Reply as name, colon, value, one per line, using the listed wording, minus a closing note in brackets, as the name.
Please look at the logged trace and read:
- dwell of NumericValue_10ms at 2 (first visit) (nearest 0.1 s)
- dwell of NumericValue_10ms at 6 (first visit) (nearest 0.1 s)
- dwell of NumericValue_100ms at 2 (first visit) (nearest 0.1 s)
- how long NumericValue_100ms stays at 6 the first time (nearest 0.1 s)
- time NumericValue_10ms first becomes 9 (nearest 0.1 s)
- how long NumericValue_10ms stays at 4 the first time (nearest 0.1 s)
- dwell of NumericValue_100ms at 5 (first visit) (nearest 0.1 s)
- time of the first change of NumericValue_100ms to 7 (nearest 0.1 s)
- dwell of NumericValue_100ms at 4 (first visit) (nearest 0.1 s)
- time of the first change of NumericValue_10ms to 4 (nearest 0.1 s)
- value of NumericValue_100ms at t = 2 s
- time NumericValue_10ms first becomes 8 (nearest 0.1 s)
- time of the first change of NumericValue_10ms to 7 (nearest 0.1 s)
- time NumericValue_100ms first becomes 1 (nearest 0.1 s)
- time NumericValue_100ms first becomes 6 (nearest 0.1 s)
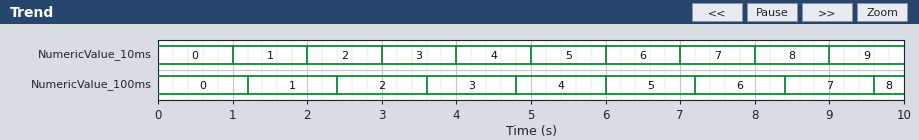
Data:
dwell of NumericValue_10ms at 2 (first visit): 1.0 s
dwell of NumericValue_10ms at 6 (first visit): 1.0 s
dwell of NumericValue_100ms at 2 (first visit): 1.2 s
how long NumericValue_100ms stays at 6 the first time: 1.2 s
time NumericValue_10ms first becomes 9: 9.0 s
how long NumericValue_10ms stays at 4 the first time: 1.0 s
dwell of NumericValue_100ms at 5 (first visit): 1.2 s
time of the first change of NumericValue_100ms to 7: 8.4 s
dwell of NumericValue_100ms at 4 (first visit): 1.2 s
time of the first change of NumericValue_10ms to 4: 4.0 s
value of NumericValue_100ms at t = 2 s: 1
time NumericValue_10ms first becomes 8: 8.0 s
time of the first change of NumericValue_10ms to 7: 7.0 s
time NumericValue_100ms first becomes 1: 1.2 s
time NumericValue_100ms first becomes 6: 7.2 s
